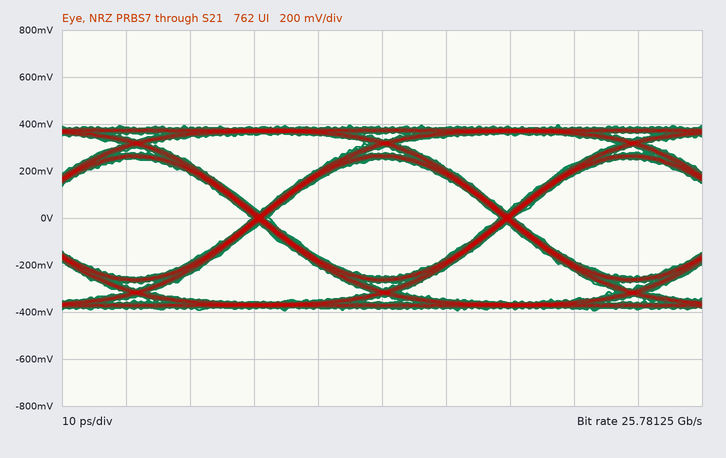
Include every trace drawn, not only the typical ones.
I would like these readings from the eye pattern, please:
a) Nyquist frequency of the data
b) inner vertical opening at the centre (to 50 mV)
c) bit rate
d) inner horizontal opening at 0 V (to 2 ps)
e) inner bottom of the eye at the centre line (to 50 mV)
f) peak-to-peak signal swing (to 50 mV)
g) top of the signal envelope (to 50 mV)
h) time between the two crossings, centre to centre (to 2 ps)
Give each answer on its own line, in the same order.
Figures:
12.89062 GHz
500 mV
25.78125 Gb/s
36 ps
-250 mV
800 mV
400 mV
38 ps
